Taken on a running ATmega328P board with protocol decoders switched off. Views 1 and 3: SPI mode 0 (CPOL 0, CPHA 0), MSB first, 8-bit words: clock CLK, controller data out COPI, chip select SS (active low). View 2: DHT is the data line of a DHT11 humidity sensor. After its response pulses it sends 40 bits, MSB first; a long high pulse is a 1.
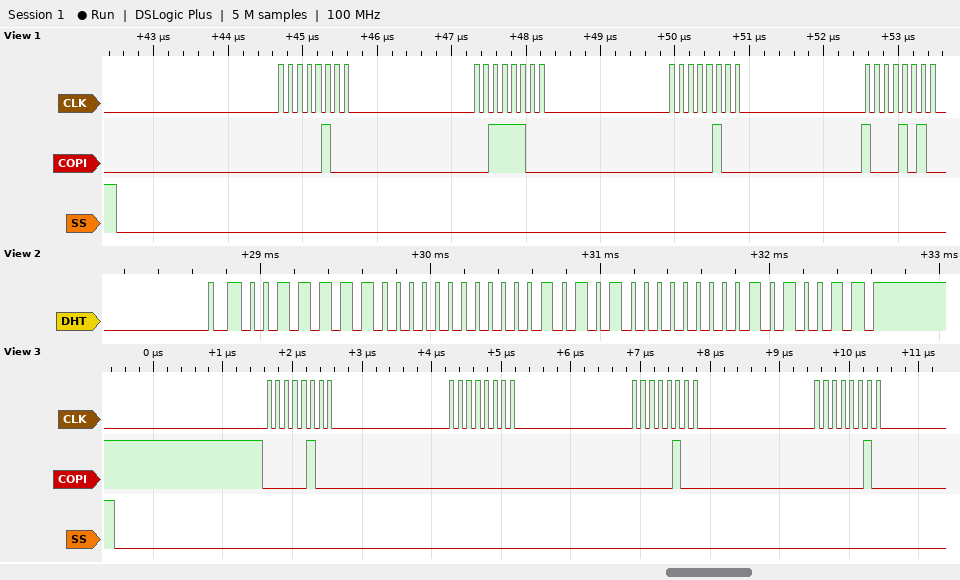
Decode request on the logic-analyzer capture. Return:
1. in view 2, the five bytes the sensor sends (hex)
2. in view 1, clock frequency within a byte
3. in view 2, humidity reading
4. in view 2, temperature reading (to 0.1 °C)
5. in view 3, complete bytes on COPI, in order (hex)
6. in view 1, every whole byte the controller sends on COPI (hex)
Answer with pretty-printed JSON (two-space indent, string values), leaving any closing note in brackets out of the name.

{
  "in view 2, the five bytes the sensor sends": "3E 00 15 00 53",
  "in view 1, clock frequency within a byte": "8 MHz",
  "in view 2, humidity reading": "62 %",
  "in view 2, temperature reading": "21.0 °C",
  "in view 3, complete bytes on COPI, in order": "0x04 0x00 0x04 0x02",
  "in view 1, every whole byte the controller sends on COPI": "04 3C 04 8A"
}
